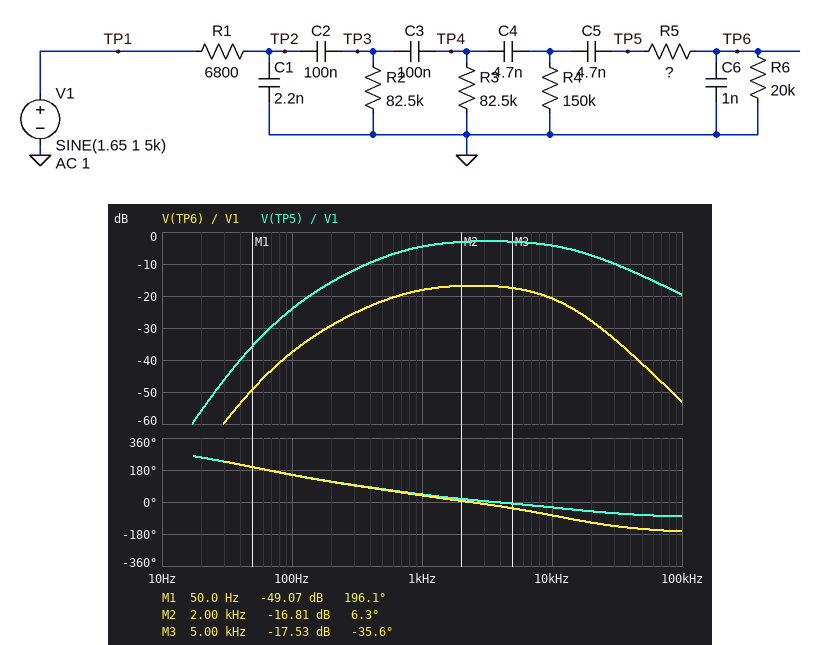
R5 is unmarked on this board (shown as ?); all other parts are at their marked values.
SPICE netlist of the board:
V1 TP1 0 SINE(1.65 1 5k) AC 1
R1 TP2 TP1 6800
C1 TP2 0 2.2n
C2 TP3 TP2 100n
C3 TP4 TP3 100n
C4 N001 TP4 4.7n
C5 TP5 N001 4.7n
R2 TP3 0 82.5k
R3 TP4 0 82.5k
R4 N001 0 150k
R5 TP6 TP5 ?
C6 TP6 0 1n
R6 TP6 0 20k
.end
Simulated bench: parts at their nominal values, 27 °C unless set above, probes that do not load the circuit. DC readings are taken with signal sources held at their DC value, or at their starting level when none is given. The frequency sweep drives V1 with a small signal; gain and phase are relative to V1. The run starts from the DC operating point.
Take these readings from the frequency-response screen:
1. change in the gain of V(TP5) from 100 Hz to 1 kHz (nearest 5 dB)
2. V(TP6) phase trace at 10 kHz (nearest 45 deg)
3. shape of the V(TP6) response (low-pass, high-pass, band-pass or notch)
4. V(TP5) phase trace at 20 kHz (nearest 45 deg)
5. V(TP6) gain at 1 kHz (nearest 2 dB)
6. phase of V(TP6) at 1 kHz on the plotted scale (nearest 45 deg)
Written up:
20 dB
-90 deg
band-pass
-45 deg
-18 dB
45 deg
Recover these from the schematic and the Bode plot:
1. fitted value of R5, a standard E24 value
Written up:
75 kΩ
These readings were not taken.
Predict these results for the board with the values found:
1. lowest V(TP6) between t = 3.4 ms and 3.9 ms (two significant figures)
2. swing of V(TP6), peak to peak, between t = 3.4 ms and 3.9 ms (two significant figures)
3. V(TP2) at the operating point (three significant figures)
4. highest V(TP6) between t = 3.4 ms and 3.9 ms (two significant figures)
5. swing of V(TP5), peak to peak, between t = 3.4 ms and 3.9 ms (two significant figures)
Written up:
-130 mV
270 mV
1.65 V
130 mV
1.4 V
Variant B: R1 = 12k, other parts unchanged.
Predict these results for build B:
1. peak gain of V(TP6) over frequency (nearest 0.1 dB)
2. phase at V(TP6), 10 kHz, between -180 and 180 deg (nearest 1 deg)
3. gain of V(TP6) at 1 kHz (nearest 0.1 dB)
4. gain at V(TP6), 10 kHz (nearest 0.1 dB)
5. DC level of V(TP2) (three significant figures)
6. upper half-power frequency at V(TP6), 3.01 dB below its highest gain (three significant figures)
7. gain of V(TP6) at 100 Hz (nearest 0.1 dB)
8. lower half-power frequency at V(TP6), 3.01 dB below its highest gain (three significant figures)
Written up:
-18.3 dB
-87 deg
-19.4 dB
-23.8 dB
1.65 V
7.17 kHz
-38.3 dB
629 Hz
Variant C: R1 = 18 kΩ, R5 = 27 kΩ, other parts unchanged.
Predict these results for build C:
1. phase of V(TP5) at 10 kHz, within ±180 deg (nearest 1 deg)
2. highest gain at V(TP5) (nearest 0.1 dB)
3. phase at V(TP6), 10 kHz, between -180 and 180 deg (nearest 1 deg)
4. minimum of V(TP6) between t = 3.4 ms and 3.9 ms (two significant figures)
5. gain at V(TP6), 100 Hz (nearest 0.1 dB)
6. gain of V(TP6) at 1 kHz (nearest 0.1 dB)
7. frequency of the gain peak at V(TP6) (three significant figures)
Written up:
-42 deg
-7.9 dB
-78 deg
-150 mV
-38.7 dB
-17.7 dB
2.62 kHz
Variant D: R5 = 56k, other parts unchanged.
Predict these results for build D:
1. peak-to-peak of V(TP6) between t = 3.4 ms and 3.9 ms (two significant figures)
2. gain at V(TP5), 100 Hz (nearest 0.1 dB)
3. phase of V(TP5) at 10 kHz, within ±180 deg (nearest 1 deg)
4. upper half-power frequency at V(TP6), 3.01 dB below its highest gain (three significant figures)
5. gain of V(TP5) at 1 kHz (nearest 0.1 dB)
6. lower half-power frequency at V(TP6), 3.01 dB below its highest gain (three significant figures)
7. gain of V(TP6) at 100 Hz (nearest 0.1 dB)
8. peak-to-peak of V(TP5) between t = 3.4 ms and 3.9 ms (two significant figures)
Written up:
330 mV
-25.8 dB
-29 deg
9.09 kHz
-5.4 dB
784 Hz
-37.4 dB
1.4 V
